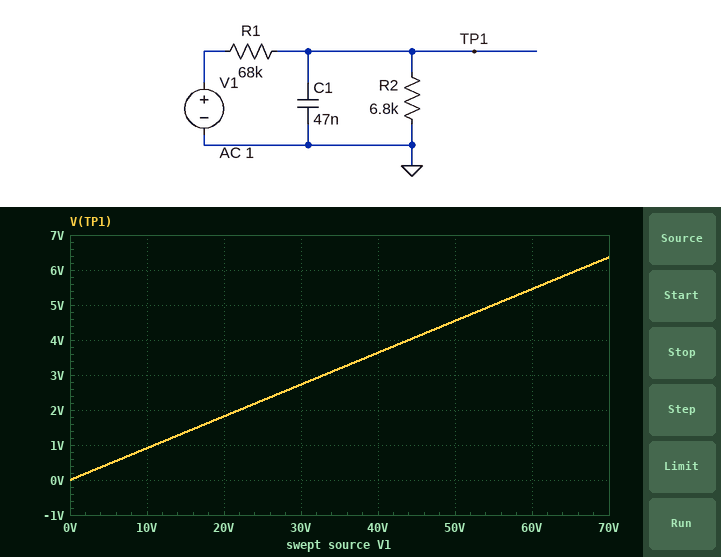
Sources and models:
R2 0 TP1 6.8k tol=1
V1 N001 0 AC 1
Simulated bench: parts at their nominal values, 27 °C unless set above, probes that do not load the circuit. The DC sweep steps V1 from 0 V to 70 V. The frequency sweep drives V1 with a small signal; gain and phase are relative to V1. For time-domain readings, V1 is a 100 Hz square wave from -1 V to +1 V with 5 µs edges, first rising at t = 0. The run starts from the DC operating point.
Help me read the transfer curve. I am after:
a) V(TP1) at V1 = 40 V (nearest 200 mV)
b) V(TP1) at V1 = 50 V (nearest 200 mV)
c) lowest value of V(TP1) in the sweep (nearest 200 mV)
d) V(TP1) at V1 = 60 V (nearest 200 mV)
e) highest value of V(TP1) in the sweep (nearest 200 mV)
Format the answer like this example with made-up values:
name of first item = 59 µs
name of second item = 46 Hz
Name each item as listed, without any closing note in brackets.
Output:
V(TP1) at V1 = 40 V = 3.6 V
V(TP1) at V1 = 50 V = 4.6 V
lowest value of V(TP1) in the sweep = 0 V
V(TP1) at V1 = 60 V = 5.4 V
highest value of V(TP1) in the sweep = 6.4 V
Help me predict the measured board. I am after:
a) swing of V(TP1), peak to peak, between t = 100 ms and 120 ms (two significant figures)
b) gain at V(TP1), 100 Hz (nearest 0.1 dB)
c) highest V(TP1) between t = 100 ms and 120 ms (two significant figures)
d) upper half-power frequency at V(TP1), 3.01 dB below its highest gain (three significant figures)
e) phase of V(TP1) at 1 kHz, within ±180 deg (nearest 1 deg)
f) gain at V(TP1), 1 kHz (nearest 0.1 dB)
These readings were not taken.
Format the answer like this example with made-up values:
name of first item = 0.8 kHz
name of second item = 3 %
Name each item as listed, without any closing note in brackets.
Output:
swing of V(TP1), peak to peak, between t = 100 ms and 120 ms = 180 mV
gain at V(TP1), 100 Hz = -21.0 dB
highest V(TP1) between t = 100 ms and 120 ms = 91 mV
upper half-power frequency at V(TP1), 3.01 dB below its highest gain = 548 Hz
phase of V(TP1) at 1 kHz, within ±180 deg = -61 deg
gain at V(TP1), 1 kHz = -27.2 dB
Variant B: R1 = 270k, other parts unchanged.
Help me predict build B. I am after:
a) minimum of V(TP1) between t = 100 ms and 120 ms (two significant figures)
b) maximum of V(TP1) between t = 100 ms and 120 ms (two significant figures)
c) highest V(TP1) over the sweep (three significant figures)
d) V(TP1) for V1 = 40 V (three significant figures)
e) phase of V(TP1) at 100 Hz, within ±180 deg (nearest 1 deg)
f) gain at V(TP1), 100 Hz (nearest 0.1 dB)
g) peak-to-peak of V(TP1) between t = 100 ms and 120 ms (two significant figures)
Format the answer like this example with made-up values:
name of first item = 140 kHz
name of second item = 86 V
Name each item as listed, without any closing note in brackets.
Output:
minimum of V(TP1) between t = 100 ms and 120 ms = -25 mV
maximum of V(TP1) between t = 100 ms and 120 ms = 25 mV
highest V(TP1) over the sweep = 1.72 V
V(TP1) for V1 = 40 V = 983 mV
phase of V(TP1) at 100 Hz, within ±180 deg = -11 deg
gain at V(TP1), 100 Hz = -32.4 dB
peak-to-peak of V(TP1) between t = 100 ms and 120 ms = 49 mV
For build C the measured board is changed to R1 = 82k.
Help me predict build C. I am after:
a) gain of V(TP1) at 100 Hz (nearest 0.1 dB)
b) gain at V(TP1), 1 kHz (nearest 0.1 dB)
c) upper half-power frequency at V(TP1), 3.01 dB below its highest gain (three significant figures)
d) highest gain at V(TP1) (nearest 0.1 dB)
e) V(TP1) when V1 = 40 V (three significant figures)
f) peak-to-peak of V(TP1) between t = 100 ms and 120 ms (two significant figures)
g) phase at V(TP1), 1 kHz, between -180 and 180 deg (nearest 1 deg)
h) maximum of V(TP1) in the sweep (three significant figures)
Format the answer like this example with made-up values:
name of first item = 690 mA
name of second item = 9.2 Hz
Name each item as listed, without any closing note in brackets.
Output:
gain of V(TP1) at 100 Hz = -22.5 dB
gain at V(TP1), 1 kHz = -28.8 dB
upper half-power frequency at V(TP1), 3.01 dB below its highest gain = 539 Hz
highest gain at V(TP1) = -22.3 dB
V(TP1) when V1 = 40 V = 3.06 V
peak-to-peak of V(TP1) between t = 100 ms and 120 ms = 150 mV
phase at V(TP1), 1 kHz, between -180 and 180 deg = -62 deg
maximum of V(TP1) in the sweep = 5.36 V
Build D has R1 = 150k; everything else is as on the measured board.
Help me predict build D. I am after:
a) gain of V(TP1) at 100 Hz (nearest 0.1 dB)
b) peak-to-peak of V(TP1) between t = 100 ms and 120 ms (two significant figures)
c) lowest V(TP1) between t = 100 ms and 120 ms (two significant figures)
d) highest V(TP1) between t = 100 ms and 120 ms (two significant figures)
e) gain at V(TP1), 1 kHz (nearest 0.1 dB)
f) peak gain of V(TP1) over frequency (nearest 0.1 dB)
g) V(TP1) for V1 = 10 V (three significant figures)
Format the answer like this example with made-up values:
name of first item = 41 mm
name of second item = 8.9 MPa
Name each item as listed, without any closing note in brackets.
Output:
gain of V(TP1) at 100 Hz = -27.4 dB
peak-to-peak of V(TP1) between t = 100 ms and 120 ms = 87 mV
lowest V(TP1) between t = 100 ms and 120 ms = -43 mV
highest V(TP1) between t = 100 ms and 120 ms = 43 mV
gain at V(TP1), 1 kHz = -34.0 dB
peak gain of V(TP1) over frequency = -27.3 dB
V(TP1) for V1 = 10 V = 434 mV
